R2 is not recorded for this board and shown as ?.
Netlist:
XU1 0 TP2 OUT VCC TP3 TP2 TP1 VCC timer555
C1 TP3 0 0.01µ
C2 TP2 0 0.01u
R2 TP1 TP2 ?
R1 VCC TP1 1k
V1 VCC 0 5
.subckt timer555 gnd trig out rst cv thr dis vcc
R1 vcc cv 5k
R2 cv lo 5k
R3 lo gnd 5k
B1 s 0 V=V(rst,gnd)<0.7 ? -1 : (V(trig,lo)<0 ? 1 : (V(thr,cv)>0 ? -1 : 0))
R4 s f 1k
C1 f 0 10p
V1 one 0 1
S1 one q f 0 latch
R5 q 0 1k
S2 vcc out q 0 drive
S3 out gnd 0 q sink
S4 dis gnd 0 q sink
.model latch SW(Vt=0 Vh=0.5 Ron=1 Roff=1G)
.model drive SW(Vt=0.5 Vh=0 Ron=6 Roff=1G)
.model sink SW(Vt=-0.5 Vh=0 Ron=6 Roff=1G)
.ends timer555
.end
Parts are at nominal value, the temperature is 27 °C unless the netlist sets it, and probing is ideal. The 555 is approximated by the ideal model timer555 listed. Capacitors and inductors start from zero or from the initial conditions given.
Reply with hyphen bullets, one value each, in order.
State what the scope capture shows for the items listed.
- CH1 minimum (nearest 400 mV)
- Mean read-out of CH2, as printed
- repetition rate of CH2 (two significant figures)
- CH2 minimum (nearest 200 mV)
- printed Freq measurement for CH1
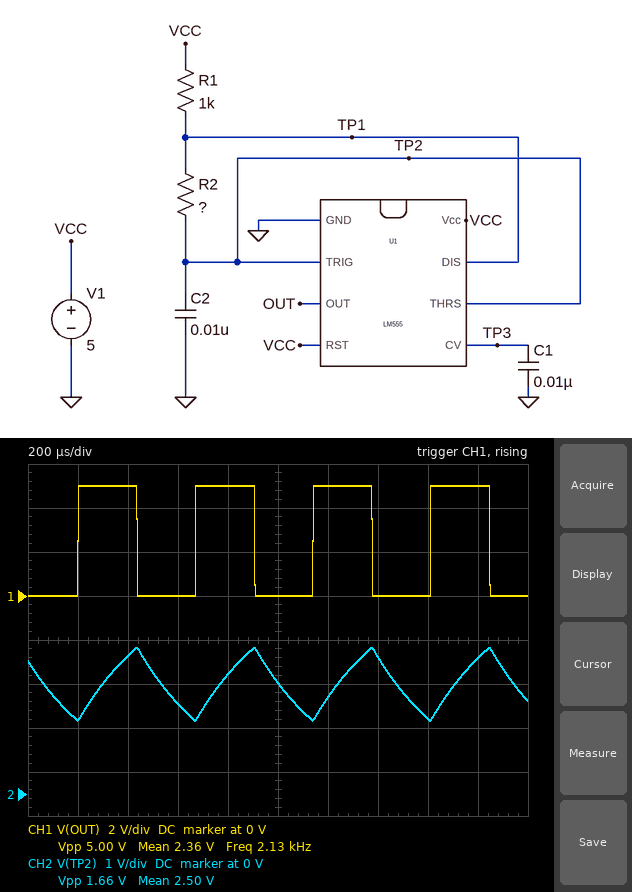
- 0 V
- 2.50 V
- 2.1 kHz
- 1.6 V
- 2.13 kHz
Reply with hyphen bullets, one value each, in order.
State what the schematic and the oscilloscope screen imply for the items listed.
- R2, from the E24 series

- 33 kΩ
